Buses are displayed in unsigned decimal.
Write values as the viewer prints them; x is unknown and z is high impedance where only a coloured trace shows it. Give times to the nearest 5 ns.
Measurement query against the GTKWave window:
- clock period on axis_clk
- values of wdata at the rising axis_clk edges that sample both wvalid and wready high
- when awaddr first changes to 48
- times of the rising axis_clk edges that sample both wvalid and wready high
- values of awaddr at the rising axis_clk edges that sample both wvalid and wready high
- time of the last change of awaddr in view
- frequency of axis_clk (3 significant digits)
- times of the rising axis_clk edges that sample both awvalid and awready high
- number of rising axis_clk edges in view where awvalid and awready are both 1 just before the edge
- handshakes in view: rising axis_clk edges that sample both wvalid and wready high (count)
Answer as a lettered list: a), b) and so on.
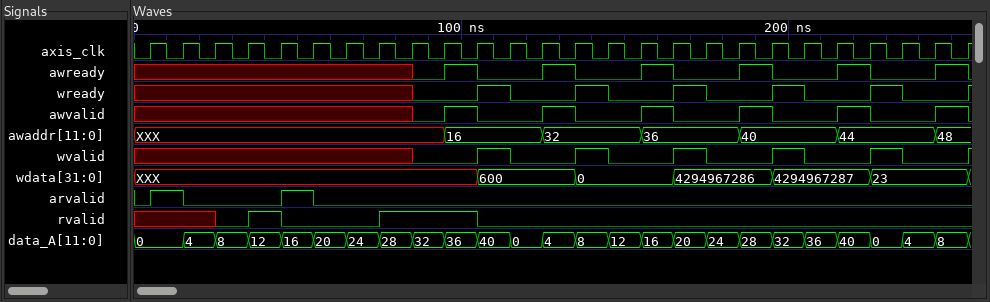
a) 10 ns
b) 600, 0, 4294967286, 4294967287, 23
c) 245 ns
d) 115 ns, 145 ns, 175 ns, 205 ns, 235 ns
e) 16, 32, 36, 40, 44
f) 245 ns
g) 100 MHz
h) 105 ns, 135 ns, 165 ns, 195 ns, 225 ns, 255 ns
i) 6
j) 5
